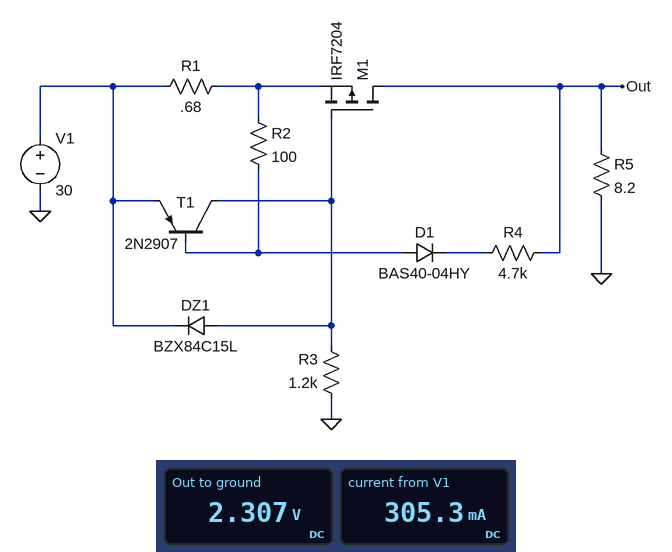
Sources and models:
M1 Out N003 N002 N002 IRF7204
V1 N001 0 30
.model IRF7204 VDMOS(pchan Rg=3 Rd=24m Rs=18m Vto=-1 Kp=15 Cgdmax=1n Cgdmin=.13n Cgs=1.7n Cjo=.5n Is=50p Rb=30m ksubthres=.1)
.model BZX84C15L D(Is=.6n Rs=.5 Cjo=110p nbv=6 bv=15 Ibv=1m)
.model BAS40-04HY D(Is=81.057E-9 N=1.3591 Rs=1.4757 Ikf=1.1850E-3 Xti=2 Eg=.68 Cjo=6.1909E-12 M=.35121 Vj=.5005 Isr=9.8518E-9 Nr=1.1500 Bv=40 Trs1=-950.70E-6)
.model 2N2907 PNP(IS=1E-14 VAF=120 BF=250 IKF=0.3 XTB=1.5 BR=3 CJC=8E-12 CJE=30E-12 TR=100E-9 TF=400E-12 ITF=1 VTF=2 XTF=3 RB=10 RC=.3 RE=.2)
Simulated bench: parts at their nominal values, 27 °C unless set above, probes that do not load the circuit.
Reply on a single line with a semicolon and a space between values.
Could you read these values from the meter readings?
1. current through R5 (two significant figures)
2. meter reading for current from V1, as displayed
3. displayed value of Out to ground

280 mA; 305.3 mA; 2.307 V
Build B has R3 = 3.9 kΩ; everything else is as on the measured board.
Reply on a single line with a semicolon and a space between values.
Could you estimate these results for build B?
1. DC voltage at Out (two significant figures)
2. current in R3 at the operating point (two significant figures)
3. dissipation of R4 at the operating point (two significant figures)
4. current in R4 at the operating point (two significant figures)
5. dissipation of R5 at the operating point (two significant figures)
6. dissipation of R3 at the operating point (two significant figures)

1.6 V; 7.4 mA; 160 mW; 5.8 mA; 310 mW; 210 mW
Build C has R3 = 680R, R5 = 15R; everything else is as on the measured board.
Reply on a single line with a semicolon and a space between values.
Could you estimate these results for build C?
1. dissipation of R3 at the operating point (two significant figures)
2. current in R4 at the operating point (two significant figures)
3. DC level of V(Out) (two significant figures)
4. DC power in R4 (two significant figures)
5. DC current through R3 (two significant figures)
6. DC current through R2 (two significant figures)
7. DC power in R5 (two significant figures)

1.2 W; 4.6 mA; 7.1 V; 100 mW; 42 mA; 4.4 mA; 3.4 W
